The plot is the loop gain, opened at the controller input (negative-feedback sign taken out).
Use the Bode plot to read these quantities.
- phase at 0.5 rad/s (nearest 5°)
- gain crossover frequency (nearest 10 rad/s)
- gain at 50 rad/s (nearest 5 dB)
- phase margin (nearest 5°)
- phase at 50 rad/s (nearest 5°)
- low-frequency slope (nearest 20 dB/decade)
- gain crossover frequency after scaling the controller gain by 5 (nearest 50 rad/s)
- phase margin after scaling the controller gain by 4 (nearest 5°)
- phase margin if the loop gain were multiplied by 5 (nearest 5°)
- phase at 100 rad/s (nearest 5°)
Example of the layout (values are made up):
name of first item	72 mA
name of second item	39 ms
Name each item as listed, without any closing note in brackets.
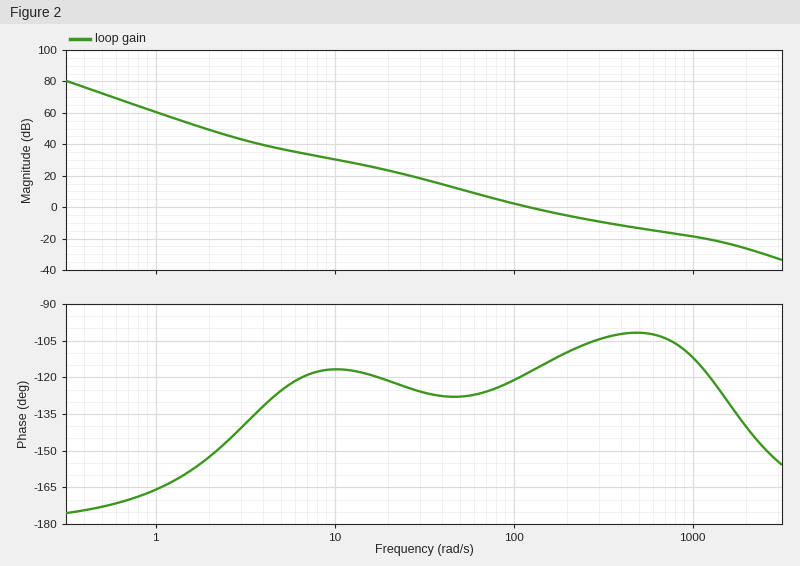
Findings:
phase at 0.5 rad/s	-175°
gain crossover frequency	120 rad/s
gain at 50 rad/s	10 dB
phase margin	60°
phase at 50 rad/s	-130°
low-frequency slope	-40 dB/decade
gain crossover frequency after scaling the controller gain by 5	550 rad/s
phase margin after scaling the controller gain by 4	80°
phase margin if the loop gain were multiplied by 5	80°
phase at 100 rad/s	-120°
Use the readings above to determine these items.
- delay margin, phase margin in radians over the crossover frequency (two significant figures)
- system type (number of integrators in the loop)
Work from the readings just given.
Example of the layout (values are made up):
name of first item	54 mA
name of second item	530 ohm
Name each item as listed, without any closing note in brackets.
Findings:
delay margin, phase margin in radians over the crossover frequency	0.0087 s
system type	2
